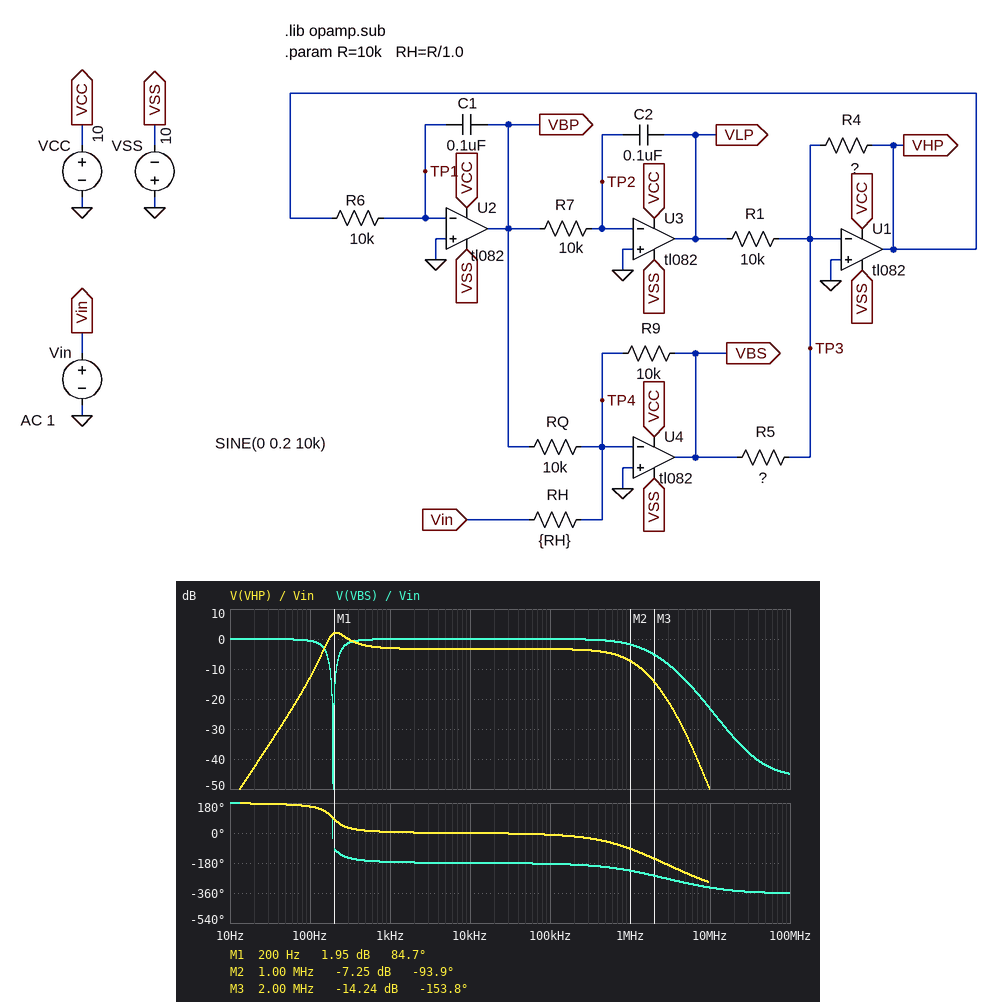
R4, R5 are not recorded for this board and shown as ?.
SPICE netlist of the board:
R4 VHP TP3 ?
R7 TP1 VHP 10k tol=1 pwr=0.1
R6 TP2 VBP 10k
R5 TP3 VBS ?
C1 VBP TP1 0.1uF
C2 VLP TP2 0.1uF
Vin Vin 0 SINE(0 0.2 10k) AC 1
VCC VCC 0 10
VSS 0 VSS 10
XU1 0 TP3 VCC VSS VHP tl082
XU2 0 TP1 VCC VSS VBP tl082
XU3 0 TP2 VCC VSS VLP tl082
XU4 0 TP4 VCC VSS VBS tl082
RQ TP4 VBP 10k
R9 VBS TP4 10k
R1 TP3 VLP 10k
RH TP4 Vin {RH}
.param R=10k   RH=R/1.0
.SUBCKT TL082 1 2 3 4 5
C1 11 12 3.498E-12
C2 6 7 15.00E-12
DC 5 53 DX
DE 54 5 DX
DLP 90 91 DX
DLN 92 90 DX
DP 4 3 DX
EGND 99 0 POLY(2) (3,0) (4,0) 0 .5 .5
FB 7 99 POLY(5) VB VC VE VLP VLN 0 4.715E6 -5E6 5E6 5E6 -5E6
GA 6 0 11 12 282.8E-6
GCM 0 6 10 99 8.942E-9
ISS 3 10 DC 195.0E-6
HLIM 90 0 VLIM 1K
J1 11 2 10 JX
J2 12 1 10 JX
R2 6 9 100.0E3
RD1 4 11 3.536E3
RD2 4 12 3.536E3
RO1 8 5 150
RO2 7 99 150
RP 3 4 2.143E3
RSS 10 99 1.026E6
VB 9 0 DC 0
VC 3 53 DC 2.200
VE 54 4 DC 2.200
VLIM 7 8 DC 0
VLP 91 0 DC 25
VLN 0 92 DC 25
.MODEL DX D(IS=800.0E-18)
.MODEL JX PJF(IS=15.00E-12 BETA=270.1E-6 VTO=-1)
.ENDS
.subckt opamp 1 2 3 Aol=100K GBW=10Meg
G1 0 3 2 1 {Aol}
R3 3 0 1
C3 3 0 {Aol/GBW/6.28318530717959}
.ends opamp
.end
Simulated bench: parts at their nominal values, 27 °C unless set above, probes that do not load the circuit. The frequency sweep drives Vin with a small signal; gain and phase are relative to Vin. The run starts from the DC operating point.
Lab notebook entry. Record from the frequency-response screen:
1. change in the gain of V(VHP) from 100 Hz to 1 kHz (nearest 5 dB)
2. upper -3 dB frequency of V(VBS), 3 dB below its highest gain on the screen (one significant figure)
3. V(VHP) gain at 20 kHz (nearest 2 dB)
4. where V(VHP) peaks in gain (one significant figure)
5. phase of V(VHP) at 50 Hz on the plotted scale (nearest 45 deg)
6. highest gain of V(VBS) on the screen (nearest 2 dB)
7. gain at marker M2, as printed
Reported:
10 dB
1 MHz
-4 dB
200 Hz
180 deg
0 dB
-7.25 dB
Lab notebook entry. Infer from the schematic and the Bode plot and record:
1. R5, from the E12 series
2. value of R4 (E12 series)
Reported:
22 kΩ
15 kΩ
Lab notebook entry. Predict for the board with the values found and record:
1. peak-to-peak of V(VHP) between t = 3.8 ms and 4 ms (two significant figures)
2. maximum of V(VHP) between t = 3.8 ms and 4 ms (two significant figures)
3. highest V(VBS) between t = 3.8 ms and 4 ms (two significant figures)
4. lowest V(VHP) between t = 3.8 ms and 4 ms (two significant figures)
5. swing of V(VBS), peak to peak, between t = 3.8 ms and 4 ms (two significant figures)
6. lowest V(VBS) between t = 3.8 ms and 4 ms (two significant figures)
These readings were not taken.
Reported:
270 mV
140 mV
200 mV
-140 mV
400 mV
-200 mV
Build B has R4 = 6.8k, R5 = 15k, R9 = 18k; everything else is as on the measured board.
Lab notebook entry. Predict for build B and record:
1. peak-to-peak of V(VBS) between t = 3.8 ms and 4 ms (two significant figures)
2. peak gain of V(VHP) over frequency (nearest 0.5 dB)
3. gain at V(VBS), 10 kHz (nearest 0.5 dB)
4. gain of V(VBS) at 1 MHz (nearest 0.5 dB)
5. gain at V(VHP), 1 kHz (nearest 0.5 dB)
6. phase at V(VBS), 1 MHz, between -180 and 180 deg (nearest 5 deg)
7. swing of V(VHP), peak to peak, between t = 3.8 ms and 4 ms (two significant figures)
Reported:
720 mV
-0.5 dB
5.0 dB
1.0 dB
-1.5 dB
120 deg
330 mV
